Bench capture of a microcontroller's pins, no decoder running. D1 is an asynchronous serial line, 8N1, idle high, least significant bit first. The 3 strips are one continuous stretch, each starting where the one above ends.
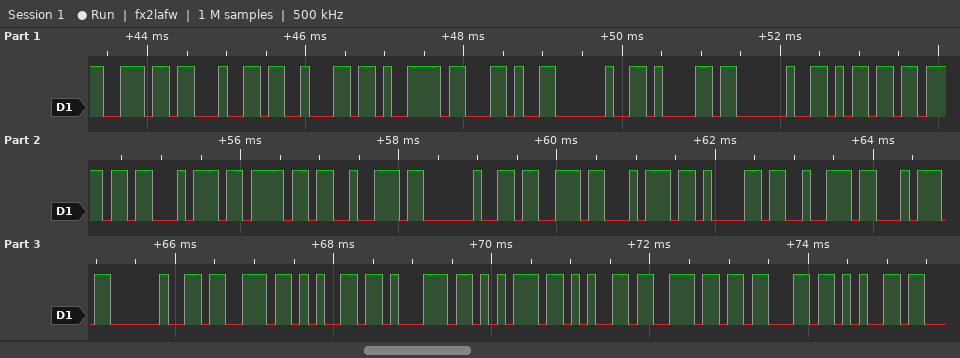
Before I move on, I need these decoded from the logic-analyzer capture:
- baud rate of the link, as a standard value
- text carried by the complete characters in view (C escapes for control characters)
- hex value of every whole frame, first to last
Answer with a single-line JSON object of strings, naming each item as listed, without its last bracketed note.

{"baud rate of the link, as a standard value": "9600 baud", "text carried by the complete characters in view": "\"ndby, a motor start sequence\"", "hex value of every whole frame, first to last": "0x6E 0x64 0x62 0x79 0x2C 0x20 0x61 0x20 0x6D 0x6F 0x74 0x6F 0x72 0x20 0x73 0x74 0x61 0x72 0x74 0x20 0x73 0x65 0x71 0x75 0x65 0x6E 0x63 0x65"}
